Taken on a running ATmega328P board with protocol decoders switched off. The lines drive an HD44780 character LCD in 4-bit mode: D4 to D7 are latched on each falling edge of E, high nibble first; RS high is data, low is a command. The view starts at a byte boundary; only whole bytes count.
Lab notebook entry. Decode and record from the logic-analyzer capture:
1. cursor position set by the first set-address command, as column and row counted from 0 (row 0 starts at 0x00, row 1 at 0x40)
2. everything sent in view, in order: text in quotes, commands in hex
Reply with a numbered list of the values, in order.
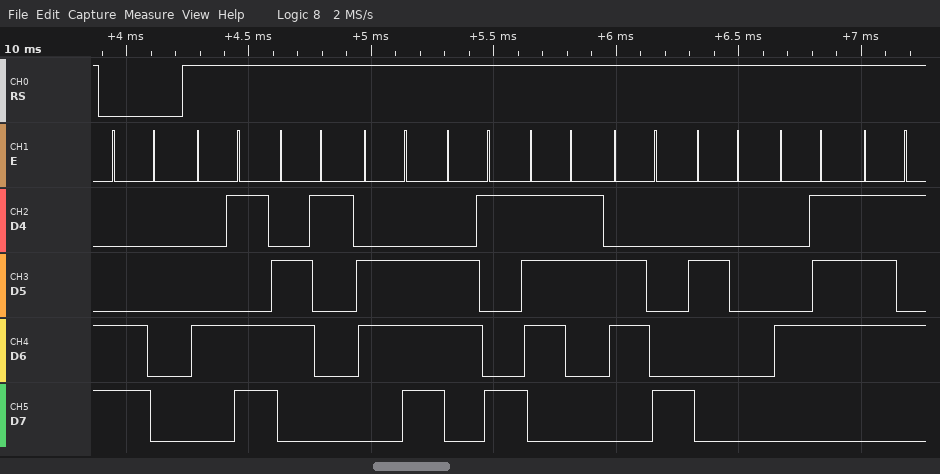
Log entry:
1. column 0, row 1
2. 0xC0 "Manish Gu"
